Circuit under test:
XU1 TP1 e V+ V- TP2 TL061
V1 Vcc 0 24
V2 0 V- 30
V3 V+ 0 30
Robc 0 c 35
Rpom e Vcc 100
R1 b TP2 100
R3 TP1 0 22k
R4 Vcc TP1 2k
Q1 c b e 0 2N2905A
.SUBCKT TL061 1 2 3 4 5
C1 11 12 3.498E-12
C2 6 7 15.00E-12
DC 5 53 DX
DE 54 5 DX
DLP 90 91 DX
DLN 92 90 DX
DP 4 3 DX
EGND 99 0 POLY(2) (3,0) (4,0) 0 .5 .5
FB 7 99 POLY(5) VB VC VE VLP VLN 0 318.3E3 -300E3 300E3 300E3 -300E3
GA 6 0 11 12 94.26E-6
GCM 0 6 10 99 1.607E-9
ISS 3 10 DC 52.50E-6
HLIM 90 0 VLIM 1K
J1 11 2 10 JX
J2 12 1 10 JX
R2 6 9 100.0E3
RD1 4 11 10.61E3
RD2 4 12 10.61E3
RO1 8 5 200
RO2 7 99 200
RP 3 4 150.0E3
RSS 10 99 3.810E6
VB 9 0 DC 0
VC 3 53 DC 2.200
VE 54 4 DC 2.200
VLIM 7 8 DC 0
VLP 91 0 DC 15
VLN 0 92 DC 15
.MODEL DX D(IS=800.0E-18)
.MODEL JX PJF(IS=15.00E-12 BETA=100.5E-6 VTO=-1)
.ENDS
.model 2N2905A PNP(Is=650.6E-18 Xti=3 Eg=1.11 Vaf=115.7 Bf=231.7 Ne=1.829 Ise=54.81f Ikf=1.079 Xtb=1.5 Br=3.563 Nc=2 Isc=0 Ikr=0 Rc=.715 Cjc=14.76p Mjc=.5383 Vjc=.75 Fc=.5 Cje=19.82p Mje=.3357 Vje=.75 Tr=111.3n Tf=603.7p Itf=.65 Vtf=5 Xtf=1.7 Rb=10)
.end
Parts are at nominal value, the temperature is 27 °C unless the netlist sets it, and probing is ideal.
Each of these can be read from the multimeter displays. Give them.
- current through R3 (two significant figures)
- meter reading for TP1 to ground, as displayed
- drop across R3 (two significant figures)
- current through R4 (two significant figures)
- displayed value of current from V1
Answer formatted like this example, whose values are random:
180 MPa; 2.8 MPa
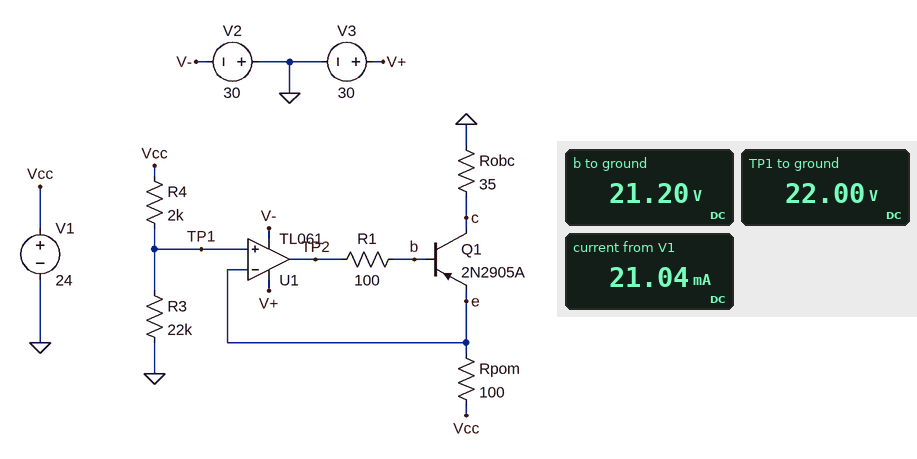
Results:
1.0 mA; 22.00 V; 22 V; 1.0 mA; 21.04 mA
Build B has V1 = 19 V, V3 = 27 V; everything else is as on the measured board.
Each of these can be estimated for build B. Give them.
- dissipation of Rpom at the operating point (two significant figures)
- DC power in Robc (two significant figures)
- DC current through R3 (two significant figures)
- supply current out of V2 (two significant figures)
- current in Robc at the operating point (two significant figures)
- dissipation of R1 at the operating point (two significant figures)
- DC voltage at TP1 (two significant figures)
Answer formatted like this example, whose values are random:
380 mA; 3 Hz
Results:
25 mW; 8.7 mW; 790 µA; 430 µA; 16 mA; 380 nW; 17 V
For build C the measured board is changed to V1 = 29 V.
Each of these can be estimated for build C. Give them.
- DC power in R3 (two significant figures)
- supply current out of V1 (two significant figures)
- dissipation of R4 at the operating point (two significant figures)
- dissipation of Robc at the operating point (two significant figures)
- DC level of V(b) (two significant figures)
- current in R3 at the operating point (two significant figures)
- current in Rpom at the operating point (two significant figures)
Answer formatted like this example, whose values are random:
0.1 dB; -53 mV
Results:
32 mW; 25 mA; 2.9 mW; 20 mW; 26 V; 1.2 mA; 24 mA
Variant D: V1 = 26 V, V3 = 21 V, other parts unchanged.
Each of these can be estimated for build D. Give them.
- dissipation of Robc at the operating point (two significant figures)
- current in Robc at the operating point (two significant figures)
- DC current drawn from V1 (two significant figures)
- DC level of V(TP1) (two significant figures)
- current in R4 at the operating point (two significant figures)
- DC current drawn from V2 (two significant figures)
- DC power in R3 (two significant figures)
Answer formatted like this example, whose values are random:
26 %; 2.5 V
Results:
110 mW; 57 mA; 58 mA; 24 V; 1.1 mA; 390 µA; 26 mW
